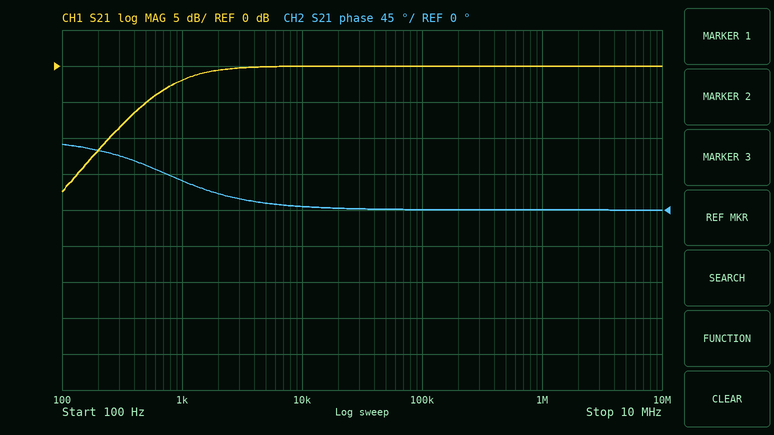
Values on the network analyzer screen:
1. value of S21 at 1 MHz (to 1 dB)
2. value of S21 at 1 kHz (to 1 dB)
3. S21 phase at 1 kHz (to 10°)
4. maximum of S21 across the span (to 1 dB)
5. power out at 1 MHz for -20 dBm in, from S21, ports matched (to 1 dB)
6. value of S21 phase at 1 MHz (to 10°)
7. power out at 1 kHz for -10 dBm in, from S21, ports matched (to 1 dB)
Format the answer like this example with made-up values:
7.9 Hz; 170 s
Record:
0 dB; -2 dB; 40°; 0 dB; -20 dBm; 0°; -12 dBm
